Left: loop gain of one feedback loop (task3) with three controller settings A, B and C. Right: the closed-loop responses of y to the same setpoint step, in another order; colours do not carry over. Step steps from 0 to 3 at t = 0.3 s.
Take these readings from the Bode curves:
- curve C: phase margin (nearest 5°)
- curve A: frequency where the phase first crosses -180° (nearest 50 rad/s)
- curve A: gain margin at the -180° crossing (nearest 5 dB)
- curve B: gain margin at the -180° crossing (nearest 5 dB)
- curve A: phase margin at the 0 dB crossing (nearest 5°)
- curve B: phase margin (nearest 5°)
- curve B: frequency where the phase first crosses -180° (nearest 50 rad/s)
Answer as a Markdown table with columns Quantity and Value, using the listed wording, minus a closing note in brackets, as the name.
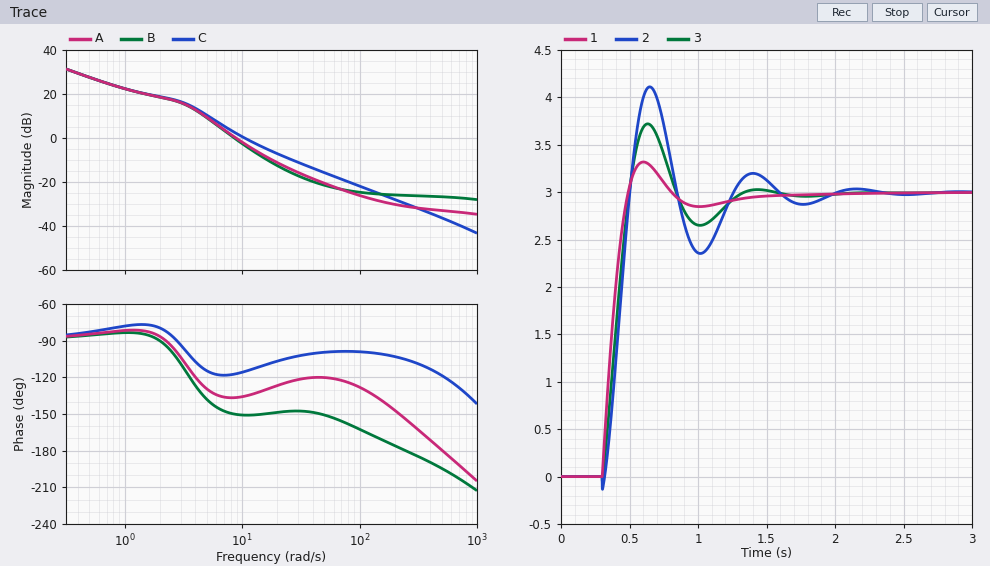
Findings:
| Quantity | Value |
|---|---|
| curve C: phase margin | 65° |
| curve A: frequency where the phase first crosses -180° | 500 rad/s |
| curve A: gain margin at the -180° crossing | 35 dB |
| curve B: gain margin at the -180° crossing | 25 dB |
| curve A: phase margin at the 0 dB crossing | 45° |
| curve B: phase margin | 30° |
| curve B: frequency where the phase first crosses -180° | 250 rad/s |
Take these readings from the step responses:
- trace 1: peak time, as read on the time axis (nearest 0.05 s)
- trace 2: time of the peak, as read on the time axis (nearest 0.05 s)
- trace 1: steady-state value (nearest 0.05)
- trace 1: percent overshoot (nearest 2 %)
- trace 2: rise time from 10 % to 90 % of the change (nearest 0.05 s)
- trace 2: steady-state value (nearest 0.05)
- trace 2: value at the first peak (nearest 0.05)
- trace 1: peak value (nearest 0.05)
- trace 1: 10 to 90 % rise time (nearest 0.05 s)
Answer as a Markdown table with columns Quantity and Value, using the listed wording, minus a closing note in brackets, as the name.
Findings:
| Quantity | Value |
|---|---|
| trace 1: peak time, as read on the time axis | 0.60 s |
| trace 2: time of the peak, as read on the time axis | 0.65 s |
| trace 1: steady-state value | 3.00 |
| trace 1: percent overshoot | 10 % |
| trace 2: rise time from 10 % to 90 % of the change | 0.15 s |
| trace 2: steady-state value | 3.00 |
| trace 2: value at the first peak | 4.10 |
| trace 1: peak value | 3.30 |
| trace 1: 10 to 90 % rise time | 0.15 s |
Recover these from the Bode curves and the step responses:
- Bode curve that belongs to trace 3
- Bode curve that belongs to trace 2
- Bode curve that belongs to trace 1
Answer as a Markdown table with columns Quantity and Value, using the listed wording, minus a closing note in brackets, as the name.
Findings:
| Quantity | Value |
|---|---|
| Bode curve that belongs to trace 3 | A |
| Bode curve that belongs to trace 2 | B |
| Bode curve that belongs to trace 1 | C |
